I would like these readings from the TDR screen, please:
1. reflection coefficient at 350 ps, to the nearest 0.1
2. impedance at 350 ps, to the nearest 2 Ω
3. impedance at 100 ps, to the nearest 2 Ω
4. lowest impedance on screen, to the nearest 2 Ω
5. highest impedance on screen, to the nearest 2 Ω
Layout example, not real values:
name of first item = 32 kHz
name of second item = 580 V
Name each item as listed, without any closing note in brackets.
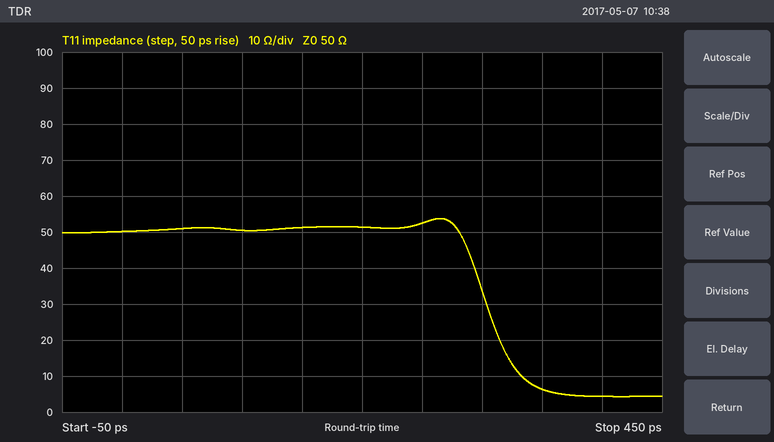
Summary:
reflection coefficient at 350 ps, to the nearest 0.1 = -0.8
impedance at 350 ps, to the nearest 2 Ω = 6 Ω
impedance at 100 ps, to the nearest 2 Ω = 50 Ω
lowest impedance on screen, to the nearest 2 Ω = 4 Ω
highest impedance on screen, to the nearest 2 Ω = 54 Ω
